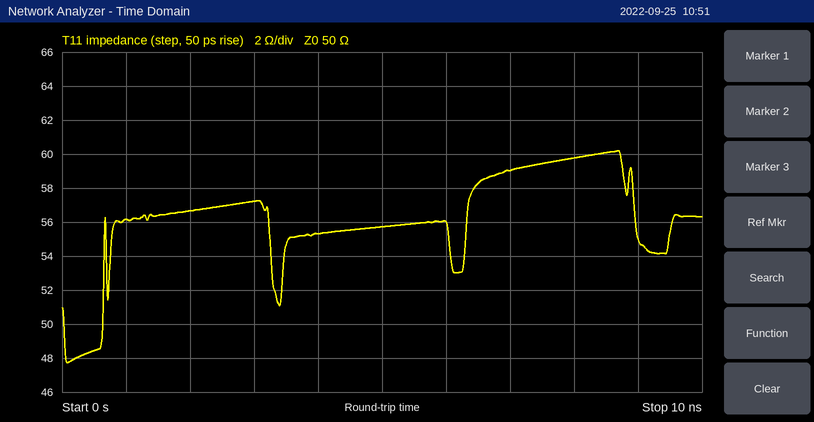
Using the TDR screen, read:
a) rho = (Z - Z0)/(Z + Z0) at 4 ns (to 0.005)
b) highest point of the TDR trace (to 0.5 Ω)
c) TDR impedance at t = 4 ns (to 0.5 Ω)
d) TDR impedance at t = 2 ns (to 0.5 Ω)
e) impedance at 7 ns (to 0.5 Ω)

+0.050
60.0 Ω
55.5 Ω
56.5 Ω
59.0 Ω
